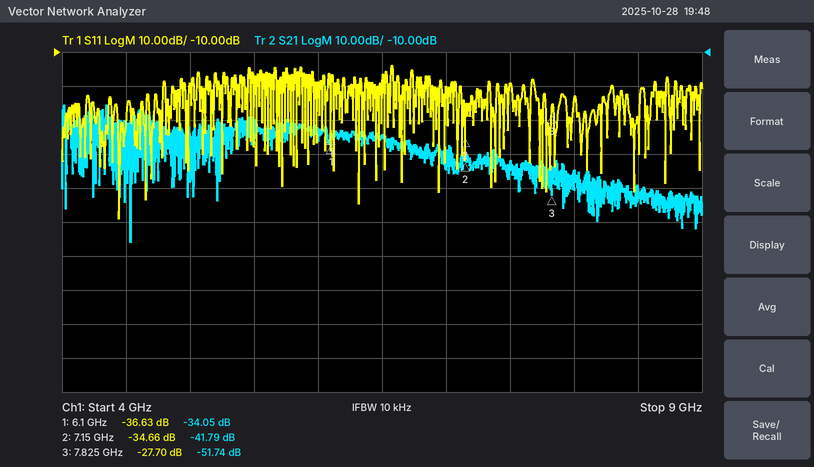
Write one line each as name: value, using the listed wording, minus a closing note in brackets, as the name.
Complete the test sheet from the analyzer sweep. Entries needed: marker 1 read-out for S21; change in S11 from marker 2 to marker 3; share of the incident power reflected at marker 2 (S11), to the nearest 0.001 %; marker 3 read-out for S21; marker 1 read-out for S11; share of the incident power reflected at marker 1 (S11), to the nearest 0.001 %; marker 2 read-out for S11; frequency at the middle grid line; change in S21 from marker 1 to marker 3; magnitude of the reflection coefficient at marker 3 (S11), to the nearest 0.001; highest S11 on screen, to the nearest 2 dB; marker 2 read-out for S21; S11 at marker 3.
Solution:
marker 1 read-out for S21: -34.05 dB
change in S11 from marker 2 to marker 3: 6.96 dB
share of the incident power reflected at marker 2 (S11), to the nearest 0.001 %: 0.034 %
marker 3 read-out for S21: -51.74 dB
marker 1 read-out for S11: -36.63 dB
share of the incident power reflected at marker 1 (S11), to the nearest 0.001 %: 0.022 %
marker 2 read-out for S11: -34.66 dB
frequency at the middle grid line: 6.5 GHz
change in S21 from marker 1 to marker 3: -17.69 dB
magnitude of the reflection coefficient at marker 3 (S11), to the nearest 0.001: 0.041
highest S11 on screen, to the nearest 2 dB: -14 dB
marker 2 read-out for S21: -41.79 dB
S11 at marker 3: -27.70 dB
